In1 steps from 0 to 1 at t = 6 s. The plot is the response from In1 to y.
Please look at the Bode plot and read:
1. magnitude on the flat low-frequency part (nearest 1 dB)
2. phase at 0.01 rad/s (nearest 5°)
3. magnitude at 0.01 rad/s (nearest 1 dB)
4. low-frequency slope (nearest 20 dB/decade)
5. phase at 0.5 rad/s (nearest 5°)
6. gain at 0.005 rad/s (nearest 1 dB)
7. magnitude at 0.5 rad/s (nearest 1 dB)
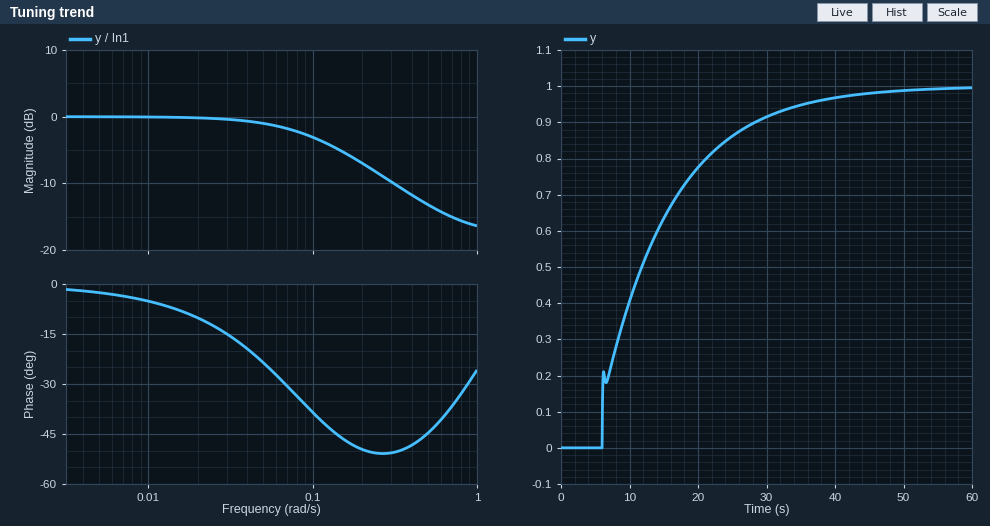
0 dB
-5°
0 dB
0 dB/decade
-45°
0 dB
-13 dB
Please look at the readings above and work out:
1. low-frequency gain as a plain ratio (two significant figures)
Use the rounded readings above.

1.0
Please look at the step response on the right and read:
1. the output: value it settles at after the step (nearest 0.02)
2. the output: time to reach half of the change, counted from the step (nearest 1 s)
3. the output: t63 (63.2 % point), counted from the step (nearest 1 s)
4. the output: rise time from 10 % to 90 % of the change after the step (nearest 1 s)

1.00
6 s
9 s
22 s
